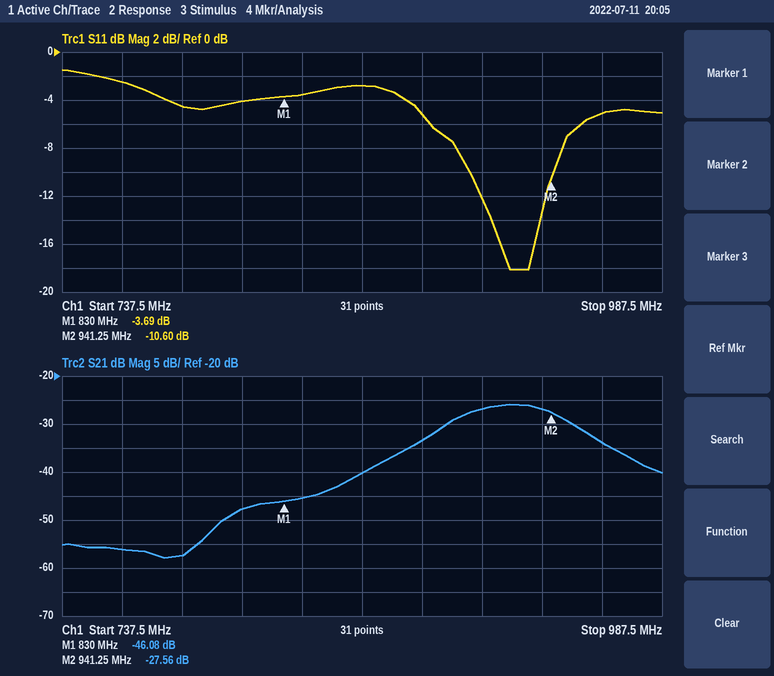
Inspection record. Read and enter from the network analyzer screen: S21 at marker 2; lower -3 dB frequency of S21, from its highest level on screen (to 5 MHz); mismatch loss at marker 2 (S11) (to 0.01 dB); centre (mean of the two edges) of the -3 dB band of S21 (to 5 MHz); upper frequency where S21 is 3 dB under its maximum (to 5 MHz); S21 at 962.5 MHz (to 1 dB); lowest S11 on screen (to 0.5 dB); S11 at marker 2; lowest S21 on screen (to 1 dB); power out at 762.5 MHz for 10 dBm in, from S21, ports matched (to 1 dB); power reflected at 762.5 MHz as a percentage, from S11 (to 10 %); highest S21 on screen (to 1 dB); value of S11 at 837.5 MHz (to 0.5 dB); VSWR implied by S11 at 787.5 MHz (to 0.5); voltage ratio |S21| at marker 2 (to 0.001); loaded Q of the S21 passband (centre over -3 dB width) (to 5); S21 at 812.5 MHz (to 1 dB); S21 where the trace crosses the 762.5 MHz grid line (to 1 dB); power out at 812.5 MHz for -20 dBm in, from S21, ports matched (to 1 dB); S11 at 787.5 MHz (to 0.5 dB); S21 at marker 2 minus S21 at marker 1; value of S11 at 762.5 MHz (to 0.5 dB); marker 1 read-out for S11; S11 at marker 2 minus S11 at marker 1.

-27.56 dB
900 MHz
0.40 dB
925 MHz
945 MHz
-34 dB
-18.0 dB
-10.60 dB
-58 dB
-46 dBm
60 %
-26 dB
-3.5 dB
4.0
0.042
20
-48 dB
-56 dB
-68 dBm
-4.5 dB
18.52 dB
-2.5 dB
-3.69 dB
-6.91 dB
